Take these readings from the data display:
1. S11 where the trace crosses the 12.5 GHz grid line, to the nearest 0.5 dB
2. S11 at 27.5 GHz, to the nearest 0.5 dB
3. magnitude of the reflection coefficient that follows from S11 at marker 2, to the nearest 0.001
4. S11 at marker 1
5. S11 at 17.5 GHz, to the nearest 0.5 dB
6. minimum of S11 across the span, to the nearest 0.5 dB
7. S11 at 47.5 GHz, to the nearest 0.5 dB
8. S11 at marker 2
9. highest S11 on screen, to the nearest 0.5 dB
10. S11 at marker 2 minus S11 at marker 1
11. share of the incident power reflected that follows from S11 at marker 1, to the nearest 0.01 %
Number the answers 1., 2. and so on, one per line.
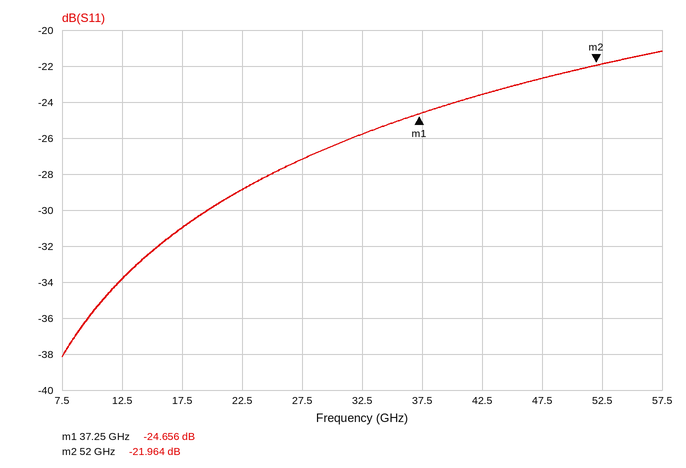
1. -34.0 dB
2. -27.0 dB
3. 0.080
4. -24.656 dB
5. -31.0 dB
6. -38.0 dB
7. -22.5 dB
8. -21.964 dB
9. -21.0 dB
10. 2.692 dB
11. 0.34 %
